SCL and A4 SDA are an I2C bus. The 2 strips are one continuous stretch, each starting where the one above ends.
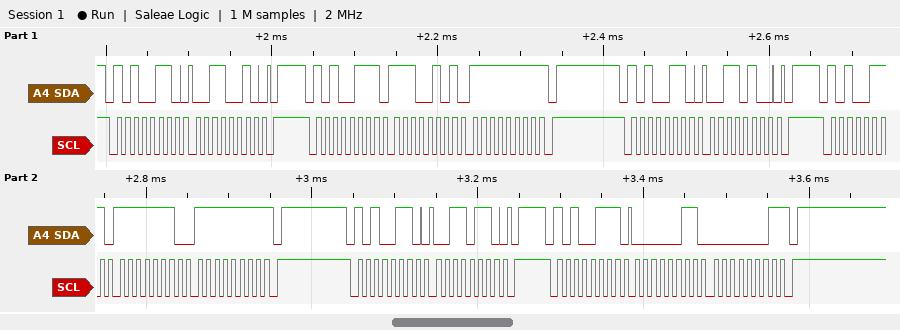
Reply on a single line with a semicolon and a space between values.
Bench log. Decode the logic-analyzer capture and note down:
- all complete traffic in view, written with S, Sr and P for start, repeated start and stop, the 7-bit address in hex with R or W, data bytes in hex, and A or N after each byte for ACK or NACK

S 53W A 32 A P S 53R A E5 A FF N P S 53W A 34 A P S 53R A FE A FF N P S 53W A 36 A P S 53R A 03 A 01 N P
